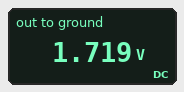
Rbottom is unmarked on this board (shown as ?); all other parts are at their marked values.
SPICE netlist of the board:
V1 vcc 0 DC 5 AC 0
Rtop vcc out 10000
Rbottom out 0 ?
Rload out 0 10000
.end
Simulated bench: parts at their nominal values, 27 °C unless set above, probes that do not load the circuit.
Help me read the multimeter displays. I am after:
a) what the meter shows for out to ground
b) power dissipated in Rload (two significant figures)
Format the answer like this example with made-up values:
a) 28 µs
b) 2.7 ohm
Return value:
a) 1.719 V
b) 300 µW
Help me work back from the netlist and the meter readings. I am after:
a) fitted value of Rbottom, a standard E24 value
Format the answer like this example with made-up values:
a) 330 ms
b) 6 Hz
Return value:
a) 11 kΩ
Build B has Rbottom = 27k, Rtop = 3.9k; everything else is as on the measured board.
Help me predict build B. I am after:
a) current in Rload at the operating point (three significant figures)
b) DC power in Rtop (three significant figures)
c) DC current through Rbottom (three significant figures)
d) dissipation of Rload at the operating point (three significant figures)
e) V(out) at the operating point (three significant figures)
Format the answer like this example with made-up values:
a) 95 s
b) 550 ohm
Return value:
a) 326 µA
b) 778 µW
c) 121 µA
d) 1.06 mW
e) 3.26 V
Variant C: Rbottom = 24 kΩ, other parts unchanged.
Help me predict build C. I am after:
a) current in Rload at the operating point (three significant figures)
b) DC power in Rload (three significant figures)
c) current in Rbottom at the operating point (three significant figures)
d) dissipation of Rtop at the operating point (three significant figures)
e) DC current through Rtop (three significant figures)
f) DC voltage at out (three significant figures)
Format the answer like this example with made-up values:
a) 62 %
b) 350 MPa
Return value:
a) 207 µA
b) 428 µW
c) 86.2 µA
d) 859 µW
e) 293 µA
f) 2.07 V
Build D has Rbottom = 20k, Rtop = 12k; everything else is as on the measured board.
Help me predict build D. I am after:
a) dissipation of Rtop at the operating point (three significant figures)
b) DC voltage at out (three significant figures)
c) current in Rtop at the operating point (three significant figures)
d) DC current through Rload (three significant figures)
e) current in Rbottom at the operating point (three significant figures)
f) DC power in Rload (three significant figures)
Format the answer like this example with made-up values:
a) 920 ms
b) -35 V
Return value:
a) 861 µW
b) 1.79 V
c) 268 µA
d) 179 µA
e) 89.3 µA
f) 319 µW
